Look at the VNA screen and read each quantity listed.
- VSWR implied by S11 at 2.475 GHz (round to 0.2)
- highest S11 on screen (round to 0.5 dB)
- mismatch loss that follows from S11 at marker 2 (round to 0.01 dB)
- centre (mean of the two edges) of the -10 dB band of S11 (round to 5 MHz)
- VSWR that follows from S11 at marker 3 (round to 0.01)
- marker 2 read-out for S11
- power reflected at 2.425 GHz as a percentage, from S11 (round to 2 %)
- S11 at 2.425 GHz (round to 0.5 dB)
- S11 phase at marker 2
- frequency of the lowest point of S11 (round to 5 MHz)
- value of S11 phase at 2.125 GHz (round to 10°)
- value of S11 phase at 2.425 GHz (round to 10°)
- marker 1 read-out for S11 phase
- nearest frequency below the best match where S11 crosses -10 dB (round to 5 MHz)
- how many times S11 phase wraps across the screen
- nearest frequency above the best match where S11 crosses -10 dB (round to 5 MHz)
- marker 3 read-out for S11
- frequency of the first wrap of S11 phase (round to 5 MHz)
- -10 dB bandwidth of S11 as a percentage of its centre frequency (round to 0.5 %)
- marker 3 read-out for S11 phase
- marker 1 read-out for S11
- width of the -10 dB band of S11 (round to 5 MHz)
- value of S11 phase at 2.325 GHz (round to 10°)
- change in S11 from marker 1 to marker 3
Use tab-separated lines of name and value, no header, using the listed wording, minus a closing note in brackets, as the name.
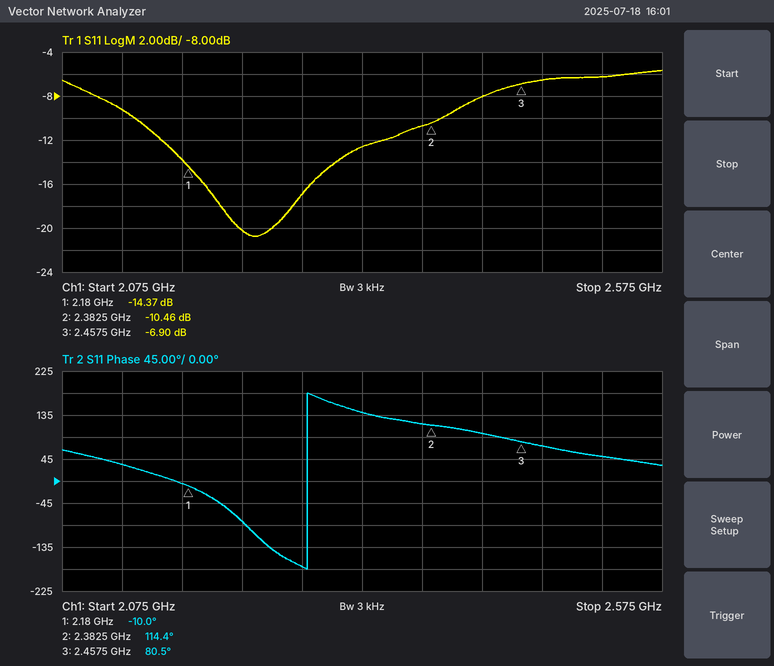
VSWR implied by S11 at 2.475 GHz	2.8
highest S11 on screen	-5.5 dB
mismatch loss that follows from S11 at marker 2	0.41 dB
centre (mean of the two edges) of the -10 dB band of S11	2.265 GHz
VSWR that follows from S11 at marker 3	2.65
marker 2 read-out for S11	-10.46 dB
power reflected at 2.425 GHz as a percentage, from S11	16 %
S11 at 2.425 GHz	-8.0 dB
S11 phase at marker 2	114.4°
frequency of the lowest point of S11	2.235 GHz
value of S11 phase at 2.125 GHz	30°
value of S11 phase at 2.425 GHz	100°
marker 1 read-out for S11 phase	-10.0°
nearest frequency below the best match where S11 crosses -10 dB	2.135 GHz
how many times S11 phase wraps across the screen	1
nearest frequency above the best match where S11 crosses -10 dB	2.390 GHz
marker 3 read-out for S11	-6.90 dB
frequency of the first wrap of S11 phase	2.280 GHz
-10 dB bandwidth of S11 as a percentage of its centre frequency	11.5 %
marker 3 read-out for S11 phase	80.5°
marker 1 read-out for S11	-14.37 dB
width of the -10 dB band of S11	255 MHz
value of S11 phase at 2.325 GHz	140°
change in S11 from marker 1 to marker 3	7.47 dB
